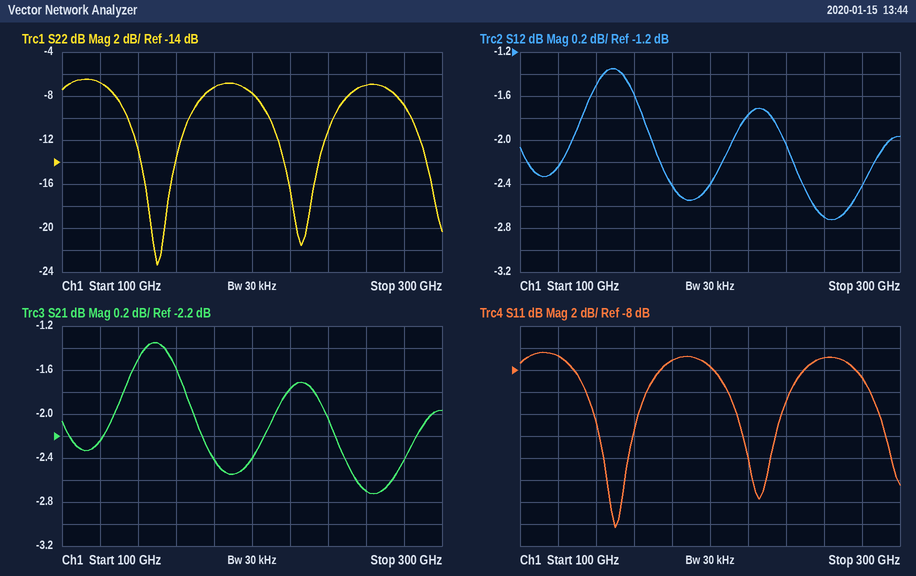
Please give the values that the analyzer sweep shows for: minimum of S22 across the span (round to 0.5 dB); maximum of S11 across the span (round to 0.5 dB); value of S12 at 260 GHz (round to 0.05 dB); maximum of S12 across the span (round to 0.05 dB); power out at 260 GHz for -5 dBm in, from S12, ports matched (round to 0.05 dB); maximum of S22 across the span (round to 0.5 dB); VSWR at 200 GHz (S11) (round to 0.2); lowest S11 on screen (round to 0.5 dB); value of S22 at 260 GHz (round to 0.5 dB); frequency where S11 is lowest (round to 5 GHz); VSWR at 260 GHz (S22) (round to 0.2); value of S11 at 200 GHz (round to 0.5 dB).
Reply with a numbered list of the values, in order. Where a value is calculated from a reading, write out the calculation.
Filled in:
1. -23.5 dB
2. -6.5 dB
3. -2.70 dB
4. -1.35 dB
5. -5 dBm + (-2.70 dB) = -7.70 dBm
6. -6.5 dB
7. |Γ| = 10^(-7.5/20) = 0.4217; VSWR = (1 + 0.4217)/(1 − 0.4217) ≈ 2.46, so 2.4 to the nearest 0.2
8. -22.5 dB
9. -7.0 dB
10. 150 GHz
11. |Γ| = 10^(-7/20) = 0.4467; VSWR = (1 + 0.4467)/(1 − 0.4467) ≈ 2.6
12. -7.5 dB
